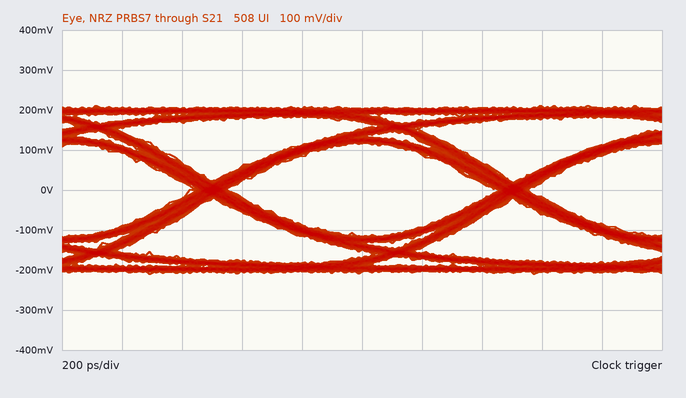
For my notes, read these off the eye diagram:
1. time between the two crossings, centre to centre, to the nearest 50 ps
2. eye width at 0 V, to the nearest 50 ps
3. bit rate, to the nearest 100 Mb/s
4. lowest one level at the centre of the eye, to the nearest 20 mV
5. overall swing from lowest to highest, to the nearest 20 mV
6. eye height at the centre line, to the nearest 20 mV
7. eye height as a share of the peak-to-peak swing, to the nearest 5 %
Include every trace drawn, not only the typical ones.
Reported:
1.00 ns
900 ps
1.0 Gb/s
120 mV
420 mV
240 mV
55 %
